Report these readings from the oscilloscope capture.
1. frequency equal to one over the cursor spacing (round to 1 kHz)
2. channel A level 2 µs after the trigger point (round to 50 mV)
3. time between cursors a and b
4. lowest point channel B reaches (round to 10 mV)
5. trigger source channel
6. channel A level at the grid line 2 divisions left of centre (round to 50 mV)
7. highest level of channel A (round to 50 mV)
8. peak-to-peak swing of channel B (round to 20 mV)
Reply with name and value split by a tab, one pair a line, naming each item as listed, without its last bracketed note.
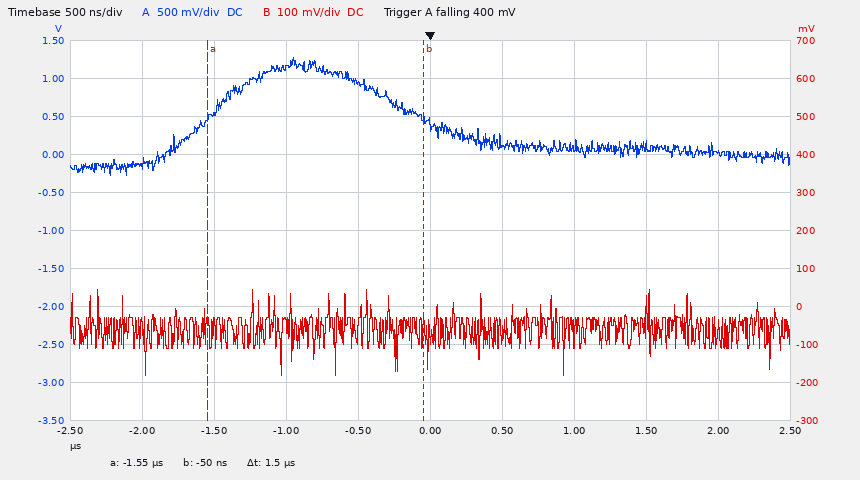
frequency equal to one over the cursor spacing	667 kHz
channel A level 2 µs after the trigger point	0 mV
time between cursors a and b	1.5 µs
lowest point channel B reaches	-180 mV
trigger source channel	channel A
channel A level at the grid line 2 divisions left of centre	1.15 V
highest level of channel A	1.30 V
peak-to-peak swing of channel B	220 mV
